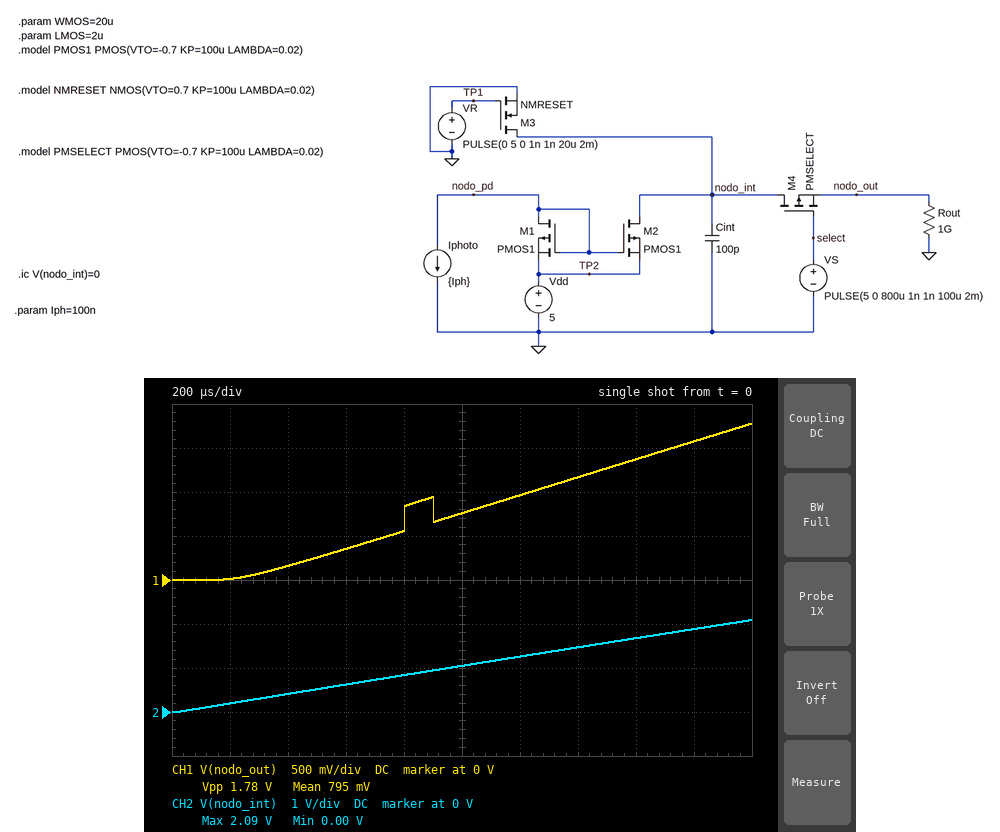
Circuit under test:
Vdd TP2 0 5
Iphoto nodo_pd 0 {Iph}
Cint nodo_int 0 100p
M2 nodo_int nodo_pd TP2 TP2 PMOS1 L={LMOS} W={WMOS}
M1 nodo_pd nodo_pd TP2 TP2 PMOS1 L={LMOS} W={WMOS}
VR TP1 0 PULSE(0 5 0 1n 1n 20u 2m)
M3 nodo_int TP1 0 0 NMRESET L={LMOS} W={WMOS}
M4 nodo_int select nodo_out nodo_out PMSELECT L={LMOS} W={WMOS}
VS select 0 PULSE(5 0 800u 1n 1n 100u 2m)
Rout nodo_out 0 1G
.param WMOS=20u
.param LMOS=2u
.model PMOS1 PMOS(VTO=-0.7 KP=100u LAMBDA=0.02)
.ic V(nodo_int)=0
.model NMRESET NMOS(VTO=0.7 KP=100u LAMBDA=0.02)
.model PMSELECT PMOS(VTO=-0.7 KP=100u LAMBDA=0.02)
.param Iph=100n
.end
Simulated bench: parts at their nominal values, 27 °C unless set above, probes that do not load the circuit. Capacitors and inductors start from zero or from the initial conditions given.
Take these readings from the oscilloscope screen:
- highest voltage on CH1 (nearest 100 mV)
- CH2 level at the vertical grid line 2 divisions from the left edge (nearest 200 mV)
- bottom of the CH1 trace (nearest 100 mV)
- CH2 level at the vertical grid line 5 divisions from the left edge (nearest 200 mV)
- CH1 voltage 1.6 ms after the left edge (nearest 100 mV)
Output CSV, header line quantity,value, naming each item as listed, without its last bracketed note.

quantity,value
highest voltage on CH1,1.8 V
CH2 level at the vertical grid line 2 divisions from the left edge,400 mV
bottom of the CH1 trace,0 V
CH2 level at the vertical grid line 5 divisions from the left edge,1.0 V
CH1 voltage 1.6 ms after the left edge,1.4 V
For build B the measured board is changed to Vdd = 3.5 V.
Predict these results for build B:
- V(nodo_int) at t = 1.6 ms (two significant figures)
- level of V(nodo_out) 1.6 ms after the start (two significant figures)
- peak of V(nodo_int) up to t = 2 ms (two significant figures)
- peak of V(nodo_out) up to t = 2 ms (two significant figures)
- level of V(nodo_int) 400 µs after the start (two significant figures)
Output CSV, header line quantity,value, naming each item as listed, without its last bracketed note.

quantity,value
V(nodo_int) at t = 1.6 ms,1.6 V
level of V(nodo_out) 1.6 ms after the start,1.3 V
peak of V(nodo_int) up to t = 2 ms,2.0 V
peak of V(nodo_out) up to t = 2 ms,1.7 V
level of V(nodo_int) 400 µs after the start,400 mV
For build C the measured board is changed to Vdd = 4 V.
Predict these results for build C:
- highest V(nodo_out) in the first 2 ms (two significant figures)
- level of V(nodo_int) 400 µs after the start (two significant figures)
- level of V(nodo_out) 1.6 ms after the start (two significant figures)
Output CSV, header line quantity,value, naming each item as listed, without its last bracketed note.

quantity,value
highest V(nodo_out) in the first 2 ms,1.7 V
level of V(nodo_int) 400 µs after the start,400 mV
level of V(nodo_out) 1.6 ms after the start,1.3 V
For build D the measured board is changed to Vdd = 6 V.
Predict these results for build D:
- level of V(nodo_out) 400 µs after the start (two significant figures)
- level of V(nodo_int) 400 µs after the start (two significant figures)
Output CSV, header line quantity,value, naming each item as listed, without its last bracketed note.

quantity,value
level of V(nodo_out) 400 µs after the start,170 mV
level of V(nodo_int) 400 µs after the start,420 mV
